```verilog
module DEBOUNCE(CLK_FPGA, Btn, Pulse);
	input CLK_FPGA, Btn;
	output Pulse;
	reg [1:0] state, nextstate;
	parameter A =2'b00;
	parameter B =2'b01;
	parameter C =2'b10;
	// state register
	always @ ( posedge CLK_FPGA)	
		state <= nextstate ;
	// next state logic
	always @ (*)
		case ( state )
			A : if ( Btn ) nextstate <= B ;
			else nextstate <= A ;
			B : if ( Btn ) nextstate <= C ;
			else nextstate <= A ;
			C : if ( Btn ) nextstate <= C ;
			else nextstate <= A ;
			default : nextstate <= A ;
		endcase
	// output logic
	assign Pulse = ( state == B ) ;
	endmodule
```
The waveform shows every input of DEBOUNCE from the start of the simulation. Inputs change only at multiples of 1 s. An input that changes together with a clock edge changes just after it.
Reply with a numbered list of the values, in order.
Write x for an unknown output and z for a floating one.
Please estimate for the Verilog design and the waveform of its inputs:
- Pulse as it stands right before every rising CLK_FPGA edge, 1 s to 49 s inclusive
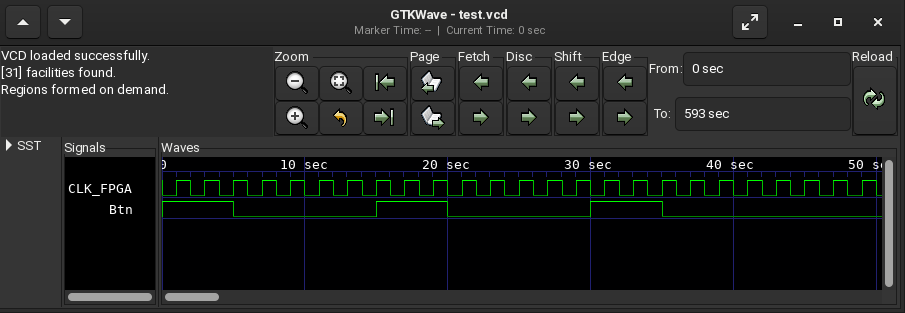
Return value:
1. x 0 1 0 0 0 0 0 0 1 0 0 0 0 0 0 1 0 0 0 0 0 0 0 0
